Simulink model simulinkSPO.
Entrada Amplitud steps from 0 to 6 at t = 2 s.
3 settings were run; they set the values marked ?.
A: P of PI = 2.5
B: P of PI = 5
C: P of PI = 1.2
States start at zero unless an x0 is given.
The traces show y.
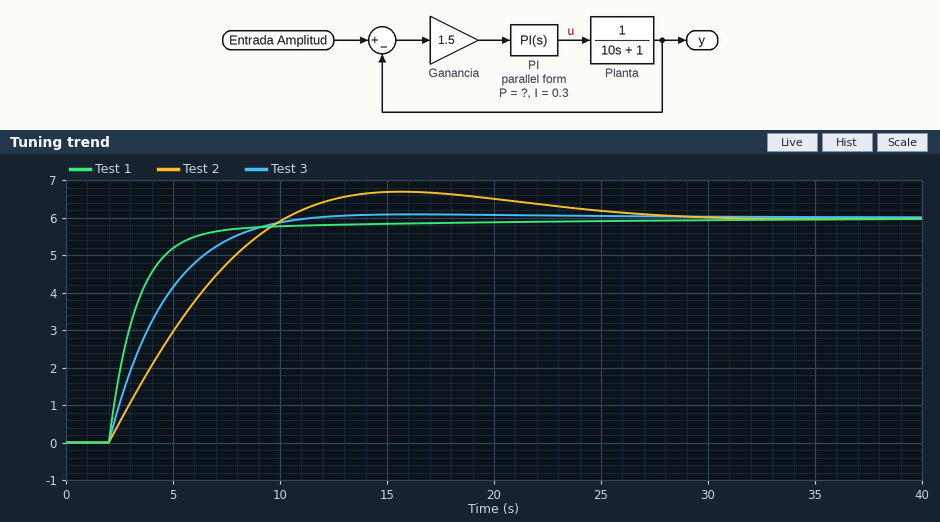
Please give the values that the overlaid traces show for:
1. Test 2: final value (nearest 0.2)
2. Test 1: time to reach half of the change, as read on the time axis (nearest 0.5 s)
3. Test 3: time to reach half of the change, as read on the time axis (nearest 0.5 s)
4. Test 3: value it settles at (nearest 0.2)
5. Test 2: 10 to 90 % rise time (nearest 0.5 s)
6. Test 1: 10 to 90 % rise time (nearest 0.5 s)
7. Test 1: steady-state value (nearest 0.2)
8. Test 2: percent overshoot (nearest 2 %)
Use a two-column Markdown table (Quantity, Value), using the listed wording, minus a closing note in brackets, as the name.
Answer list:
| Quantity | Value |
|---|---|
| Test 2: final value | 6.0 |
| Test 1: time to reach half of the change, as read on the time axis | 3.0 s |
| Test 3: time to reach half of the change, as read on the time axis | 4.0 s |
| Test 3: value it settles at | 6.0 |
| Test 2: 10 to 90 % rise time | 6.0 s |
| Test 1: 10 to 90 % rise time | 3.5 s |
| Test 1: steady-state value | 6.0 |
| Test 2: percent overshoot | 12 % |
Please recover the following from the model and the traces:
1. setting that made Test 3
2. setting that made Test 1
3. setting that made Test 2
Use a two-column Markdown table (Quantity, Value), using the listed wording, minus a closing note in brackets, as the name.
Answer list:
| Quantity | Value |
|---|---|
| setting that made Test 3 | A |
| setting that made Test 1 | B |
| setting that made Test 2 | C |
